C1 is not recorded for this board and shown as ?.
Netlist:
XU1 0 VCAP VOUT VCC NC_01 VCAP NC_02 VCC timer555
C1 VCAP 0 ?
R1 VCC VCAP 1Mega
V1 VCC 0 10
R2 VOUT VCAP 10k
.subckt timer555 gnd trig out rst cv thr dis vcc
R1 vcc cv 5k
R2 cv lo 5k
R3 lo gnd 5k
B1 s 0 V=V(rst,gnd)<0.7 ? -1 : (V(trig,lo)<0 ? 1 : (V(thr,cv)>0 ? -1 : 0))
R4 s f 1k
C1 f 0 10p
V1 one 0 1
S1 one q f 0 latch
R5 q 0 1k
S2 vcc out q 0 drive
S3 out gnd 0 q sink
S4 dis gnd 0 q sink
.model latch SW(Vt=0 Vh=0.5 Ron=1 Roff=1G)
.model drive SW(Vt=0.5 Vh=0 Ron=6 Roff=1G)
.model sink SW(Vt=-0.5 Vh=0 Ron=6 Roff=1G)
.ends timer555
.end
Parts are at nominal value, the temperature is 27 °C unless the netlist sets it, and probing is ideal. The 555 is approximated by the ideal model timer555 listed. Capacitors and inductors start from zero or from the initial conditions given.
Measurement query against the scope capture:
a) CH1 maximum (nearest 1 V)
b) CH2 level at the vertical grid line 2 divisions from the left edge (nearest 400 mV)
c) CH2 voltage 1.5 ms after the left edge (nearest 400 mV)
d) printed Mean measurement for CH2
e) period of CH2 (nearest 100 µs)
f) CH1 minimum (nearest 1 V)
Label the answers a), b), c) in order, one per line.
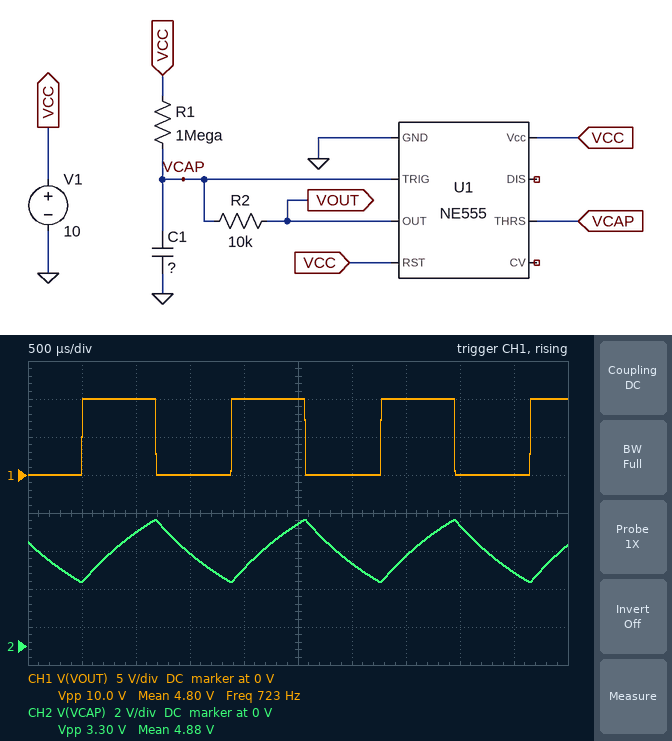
a) 10 V
b) 6.0 V
c) 4.8 V
d) 4.88 V
e) 1.4 ms
f) 0 V
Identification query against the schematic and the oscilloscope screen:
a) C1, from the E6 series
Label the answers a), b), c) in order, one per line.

a) 100 nF
